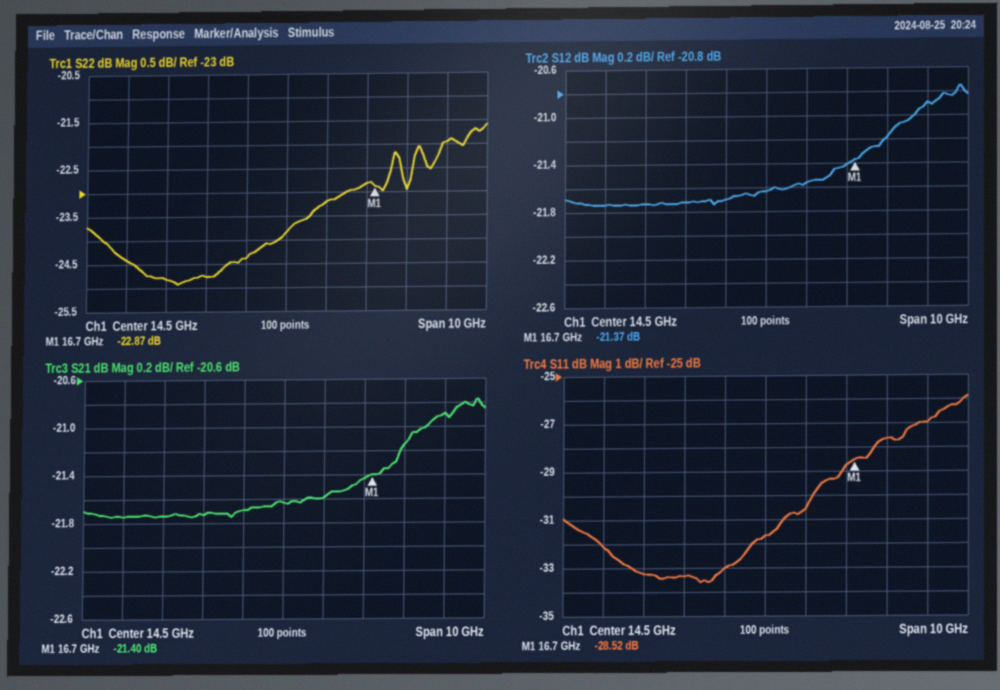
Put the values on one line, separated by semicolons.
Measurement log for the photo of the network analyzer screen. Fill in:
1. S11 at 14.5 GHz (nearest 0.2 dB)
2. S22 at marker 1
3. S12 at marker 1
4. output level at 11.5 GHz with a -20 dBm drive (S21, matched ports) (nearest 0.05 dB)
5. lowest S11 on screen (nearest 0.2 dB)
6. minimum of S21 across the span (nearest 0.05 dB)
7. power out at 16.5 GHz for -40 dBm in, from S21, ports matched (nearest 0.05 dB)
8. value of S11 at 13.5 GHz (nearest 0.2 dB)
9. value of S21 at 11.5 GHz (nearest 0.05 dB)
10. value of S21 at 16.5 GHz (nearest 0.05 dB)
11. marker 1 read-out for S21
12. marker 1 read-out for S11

-31.6 dB; -22.87 dB; -21.37 dB; -41.75 dBm; -33.6 dB; -21.75 dB; -61.45 dBm; -33.0 dB; -21.75 dB; -21.45 dB; -21.40 dB; -28.52 dB
